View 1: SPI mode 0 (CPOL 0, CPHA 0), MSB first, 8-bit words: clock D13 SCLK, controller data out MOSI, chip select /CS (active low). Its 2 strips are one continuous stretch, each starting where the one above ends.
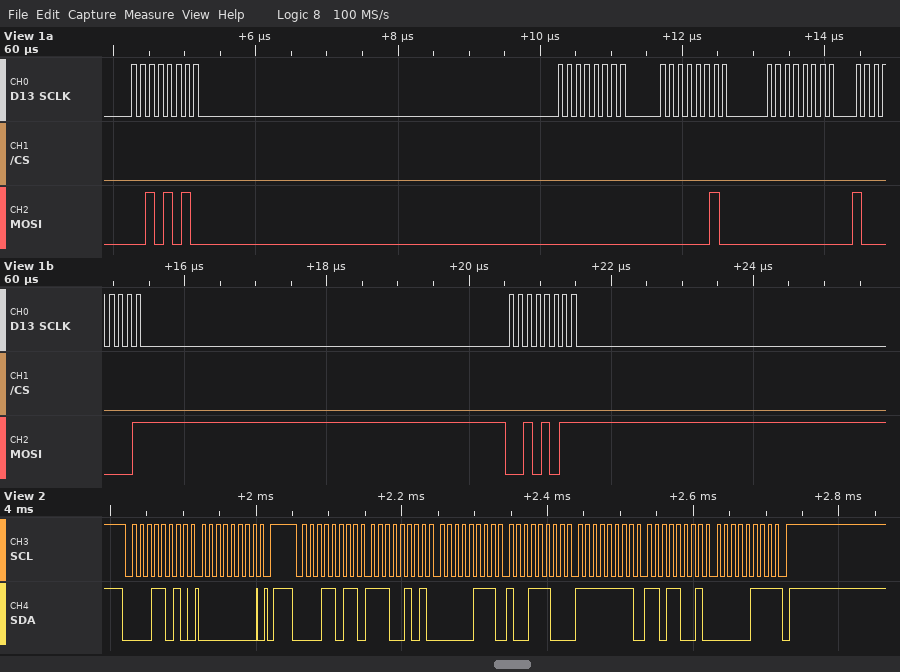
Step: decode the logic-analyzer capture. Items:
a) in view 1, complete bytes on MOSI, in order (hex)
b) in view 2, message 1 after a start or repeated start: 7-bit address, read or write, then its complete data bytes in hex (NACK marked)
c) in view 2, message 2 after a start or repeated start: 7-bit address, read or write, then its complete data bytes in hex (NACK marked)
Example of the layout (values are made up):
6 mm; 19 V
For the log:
2A 00 02 00 81 2B; 0x0D write: 00; 0x0D read: E5 07 9C FF D9 07 NACK
